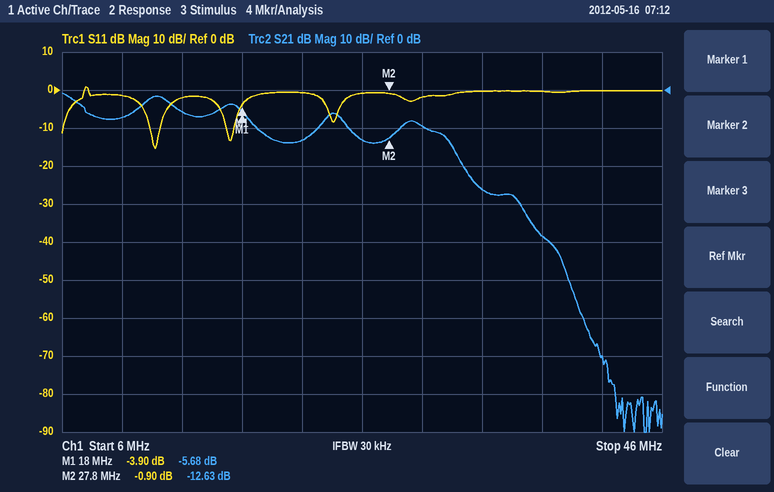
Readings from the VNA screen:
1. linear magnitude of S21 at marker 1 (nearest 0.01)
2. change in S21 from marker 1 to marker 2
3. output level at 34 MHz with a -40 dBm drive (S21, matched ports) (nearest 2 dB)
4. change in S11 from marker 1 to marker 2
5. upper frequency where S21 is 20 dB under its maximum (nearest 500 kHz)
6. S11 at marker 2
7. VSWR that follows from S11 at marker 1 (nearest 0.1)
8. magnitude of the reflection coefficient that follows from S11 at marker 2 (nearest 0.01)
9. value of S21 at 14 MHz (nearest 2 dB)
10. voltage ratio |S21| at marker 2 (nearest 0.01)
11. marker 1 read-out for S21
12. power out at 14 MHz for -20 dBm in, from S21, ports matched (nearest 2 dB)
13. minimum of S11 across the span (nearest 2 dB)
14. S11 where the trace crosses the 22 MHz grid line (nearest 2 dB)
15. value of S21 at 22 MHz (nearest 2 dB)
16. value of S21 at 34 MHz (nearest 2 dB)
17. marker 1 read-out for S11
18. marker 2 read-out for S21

0.52
-6.95 dB
-66 dBm
3.00 dB
33.0 MHz
-0.90 dB
4.5
0.90
-6 dB
0.23
-5.68 dB
-26 dBm
-16 dB
0 dB
-14 dB
-26 dB
-3.90 dB
-12.63 dB
